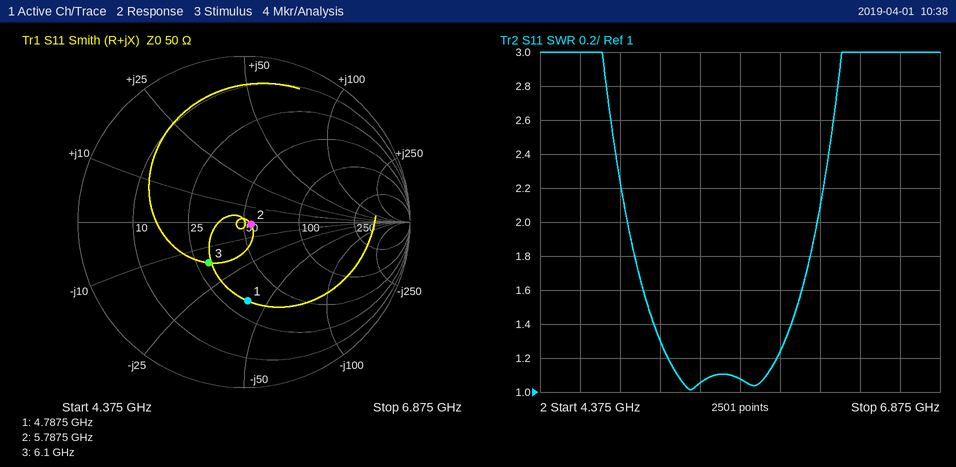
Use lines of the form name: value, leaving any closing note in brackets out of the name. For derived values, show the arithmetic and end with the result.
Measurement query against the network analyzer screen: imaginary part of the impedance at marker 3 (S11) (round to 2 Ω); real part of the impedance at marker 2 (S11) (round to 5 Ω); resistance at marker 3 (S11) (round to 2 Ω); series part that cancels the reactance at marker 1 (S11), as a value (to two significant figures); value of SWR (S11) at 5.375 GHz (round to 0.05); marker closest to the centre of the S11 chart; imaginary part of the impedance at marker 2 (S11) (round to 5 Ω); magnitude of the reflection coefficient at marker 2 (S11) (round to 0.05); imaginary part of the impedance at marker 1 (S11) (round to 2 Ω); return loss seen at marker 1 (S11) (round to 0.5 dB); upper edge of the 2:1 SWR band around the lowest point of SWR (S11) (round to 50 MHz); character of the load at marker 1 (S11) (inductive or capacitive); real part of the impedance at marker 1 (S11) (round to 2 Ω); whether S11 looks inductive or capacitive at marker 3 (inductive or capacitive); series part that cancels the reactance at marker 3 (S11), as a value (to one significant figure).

imaginary part of the impedance at marker 3 (S11): -16 Ω
real part of the impedance at marker 2 (S11): 55 Ω
resistance at marker 3 (S11): 30 Ω
series part that cancels the reactance at marker 1 (S11), as a value: L = 40 Ω/(2π × 4.7875 GHz) ≈ 1.3 nH
value of SWR (S11) at 5.375 GHz: 1.05
marker closest to the centre of the S11 chart: marker 2
imaginary part of the impedance at marker 2 (S11): 0 Ω
magnitude of the reflection coefficient at marker 2 (S11): 0.05
imaginary part of the impedance at marker 1 (S11): -40 Ω
return loss seen at marker 1 (S11): 6.5 dB
upper edge of the 2:1 SWR band around the lowest point of SWR (S11): 6.10 GHz
character of the load at marker 1 (S11): capacitive
real part of the impedance at marker 1 (S11): 32 Ω
whether S11 looks inductive or capacitive at marker 3: capacitive
series part that cancels the reactance at marker 3 (S11), as a value: L = 16 Ω/(2π × 6.1 GHz) ≈ 417 pH, so 400 pH to one significant figure
